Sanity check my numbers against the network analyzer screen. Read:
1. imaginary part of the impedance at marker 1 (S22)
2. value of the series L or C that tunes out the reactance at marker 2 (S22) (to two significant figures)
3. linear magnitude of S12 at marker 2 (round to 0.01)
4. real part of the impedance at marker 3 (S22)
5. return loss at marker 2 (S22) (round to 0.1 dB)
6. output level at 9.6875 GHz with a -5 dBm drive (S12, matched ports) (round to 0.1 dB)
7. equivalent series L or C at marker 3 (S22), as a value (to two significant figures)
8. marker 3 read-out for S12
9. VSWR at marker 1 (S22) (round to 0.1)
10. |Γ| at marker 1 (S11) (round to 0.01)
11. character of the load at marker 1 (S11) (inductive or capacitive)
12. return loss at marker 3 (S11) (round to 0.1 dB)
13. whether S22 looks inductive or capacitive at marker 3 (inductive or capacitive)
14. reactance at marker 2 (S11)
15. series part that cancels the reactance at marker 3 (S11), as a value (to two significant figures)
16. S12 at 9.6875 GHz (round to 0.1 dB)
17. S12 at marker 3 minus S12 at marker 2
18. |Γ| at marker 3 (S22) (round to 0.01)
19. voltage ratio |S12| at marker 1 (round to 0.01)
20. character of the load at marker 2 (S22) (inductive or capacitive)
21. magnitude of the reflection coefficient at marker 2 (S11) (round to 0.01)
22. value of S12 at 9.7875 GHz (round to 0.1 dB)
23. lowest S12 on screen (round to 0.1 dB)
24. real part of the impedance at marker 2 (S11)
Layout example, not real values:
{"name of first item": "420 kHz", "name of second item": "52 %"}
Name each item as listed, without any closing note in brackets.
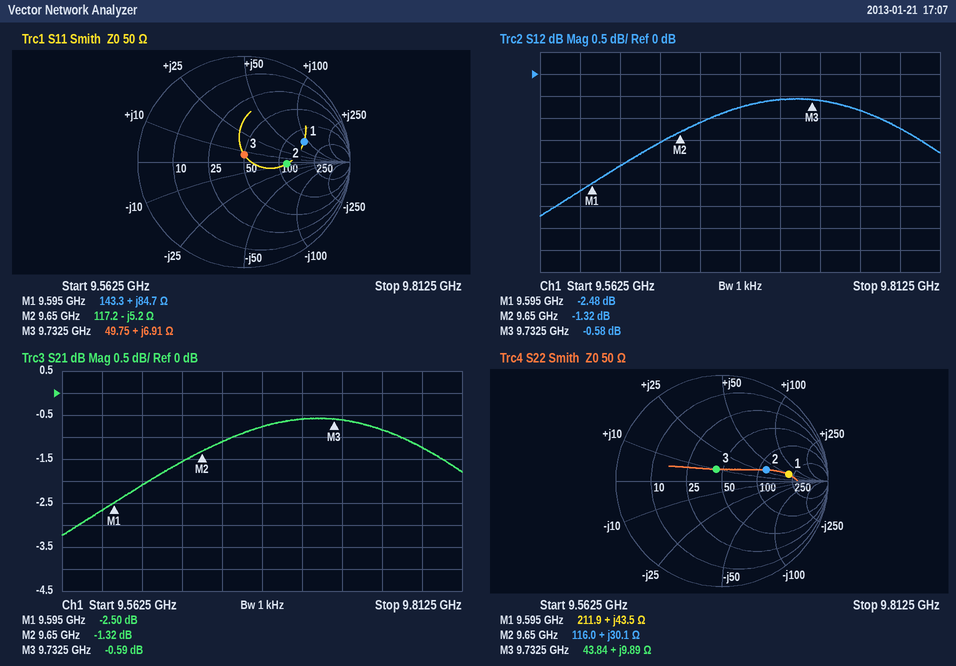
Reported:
{"imaginary part of the impedance at marker 1": "+43.5 Ω", "value of the series L or C that tunes out the reactance at marker 2 (S22)": "550 fF", "linear magnitude of S12 at marker 2": "0.86", "real part of the impedance at marker 3": "43.84 Ω", "return loss at marker 2 (S22)": "7.3 dB", "output level at 9.6875 GHz with a -5 dBm drive (S12, matched ports)": "-5.8 dBm", "equivalent series L or C at marker 3 (S22), as a value": "160 pH", "marker 3 read-out for S12": "-0.58 dB", "VSWR at marker 1 (S22)": "4.4", "|Γ| at marker 1 (S11)": "0.60", "character of the load at marker 1 (S11)": "inductive", "return loss at marker 3 (S11)": "23.2 dB", "whether S22 looks inductive or capacitive at marker 3": "inductive", "reactance at marker 2": "-5.2 Ω", "series part that cancels the reactance at marker 3 (S11), as a value": "2.4 pF", "S12 at 9.6875 GHz": "-0.8 dB", "S12 at marker 3 minus S12 at marker 2": "0.74 dB", "|Γ| at marker 3 (S22)": "0.12", "voltage ratio |S12| at marker 1": "0.75", "character of the load at marker 2 (S22)": "inductive", "magnitude of the reflection coefficient at marker 2 (S11)": "0.40", "value of S12 at 9.7875 GHz": "-1.2 dB", "lowest S12 on screen": "-3.2 dB", "real part of the impedance at marker 2": "117.2 Ω"}
